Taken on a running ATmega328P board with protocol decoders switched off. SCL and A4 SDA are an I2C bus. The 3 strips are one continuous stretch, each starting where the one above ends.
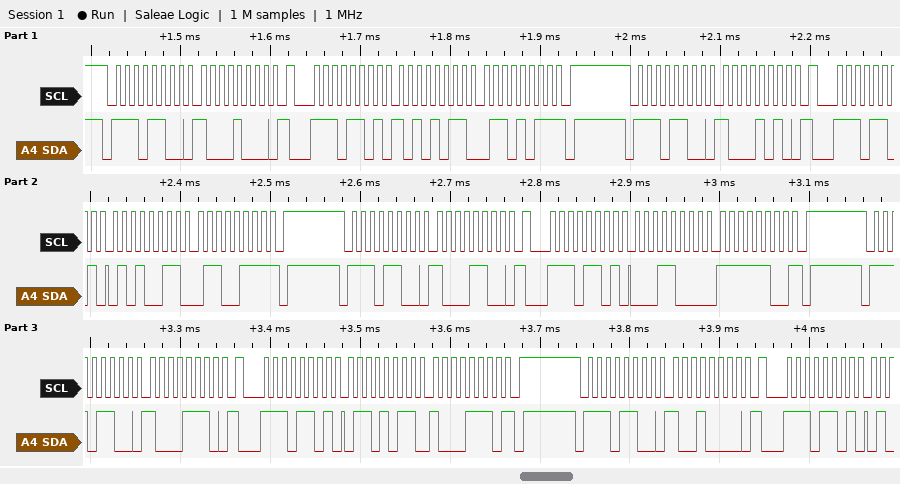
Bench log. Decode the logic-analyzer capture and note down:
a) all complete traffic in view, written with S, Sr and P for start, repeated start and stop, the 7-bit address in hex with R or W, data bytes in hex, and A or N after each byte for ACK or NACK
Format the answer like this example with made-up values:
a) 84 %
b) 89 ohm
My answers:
a) S 76W A 88 A Sr 76R A AB A 6B N P S 76W A 8A A Sr 76R A 53 A 67 N P S 76W A 8C A Sr 76R A 18 A FC N P S 76W A 8E A Sr 76R A 6B A 8E N P S 76W A 90 A Sr 76R A
